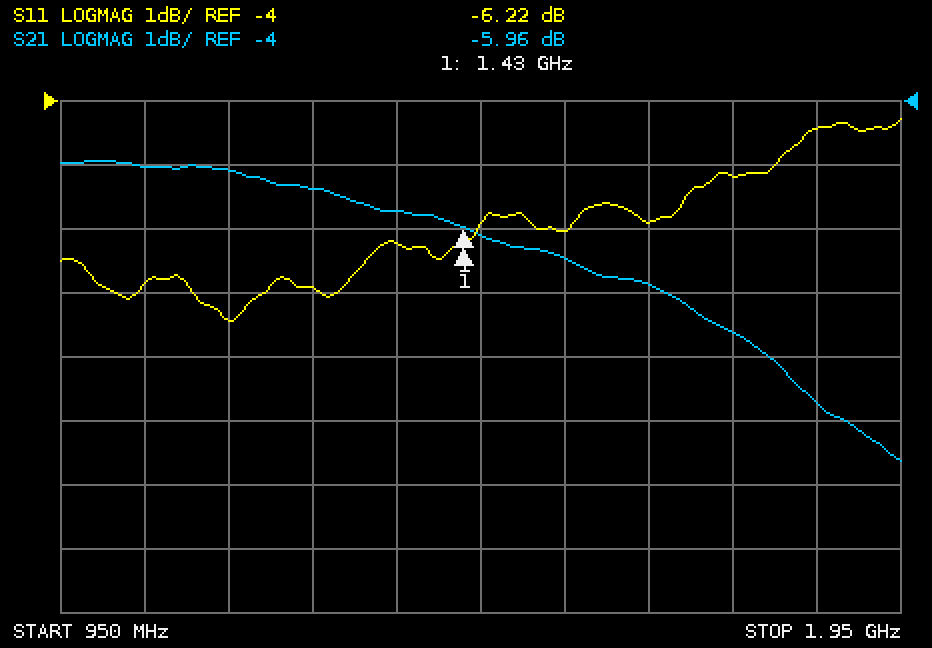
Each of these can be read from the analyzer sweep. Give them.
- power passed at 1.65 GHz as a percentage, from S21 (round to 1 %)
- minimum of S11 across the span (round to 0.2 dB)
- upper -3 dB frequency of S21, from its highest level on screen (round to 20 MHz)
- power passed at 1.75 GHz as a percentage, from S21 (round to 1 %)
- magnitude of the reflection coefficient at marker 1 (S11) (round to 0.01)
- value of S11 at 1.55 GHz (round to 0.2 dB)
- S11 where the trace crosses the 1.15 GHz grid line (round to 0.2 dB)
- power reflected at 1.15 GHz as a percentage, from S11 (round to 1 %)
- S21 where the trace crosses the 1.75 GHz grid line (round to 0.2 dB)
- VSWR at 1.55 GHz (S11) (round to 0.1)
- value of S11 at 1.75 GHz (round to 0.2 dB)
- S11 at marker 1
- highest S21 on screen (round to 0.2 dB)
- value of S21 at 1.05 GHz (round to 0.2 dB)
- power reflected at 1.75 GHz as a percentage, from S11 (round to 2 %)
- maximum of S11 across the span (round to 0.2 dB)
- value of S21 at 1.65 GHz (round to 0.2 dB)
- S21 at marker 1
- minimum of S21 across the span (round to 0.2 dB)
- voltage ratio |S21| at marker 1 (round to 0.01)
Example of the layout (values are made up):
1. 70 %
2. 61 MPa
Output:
1. 21 %
2. -7.4 dB
3. 1.78 GHz
4. 17 %
5. 0.49
6. -6.0 dB
7. -7.4 dB
8. 18 %
9. -7.6 dB
10. 3.0
11. -5.2 dB
12. -6.22 dB
13. -5.0 dB
14. -5.0 dB
15. 30 %
16. -4.2 dB
17. -6.8 dB
18. -5.96 dB
19. -9.6 dB
20. 0.50
